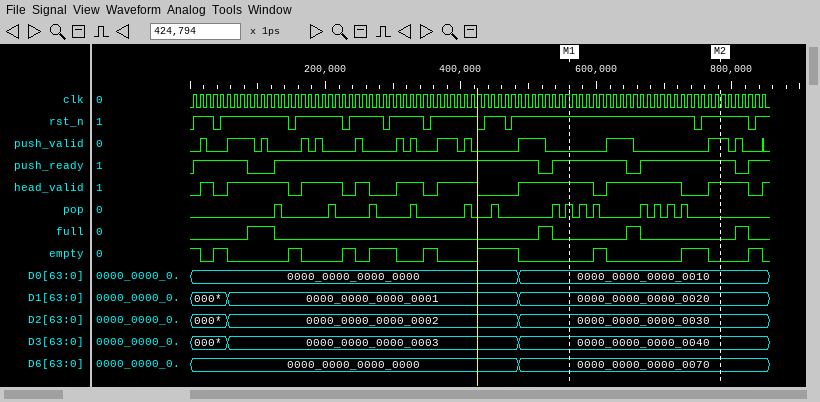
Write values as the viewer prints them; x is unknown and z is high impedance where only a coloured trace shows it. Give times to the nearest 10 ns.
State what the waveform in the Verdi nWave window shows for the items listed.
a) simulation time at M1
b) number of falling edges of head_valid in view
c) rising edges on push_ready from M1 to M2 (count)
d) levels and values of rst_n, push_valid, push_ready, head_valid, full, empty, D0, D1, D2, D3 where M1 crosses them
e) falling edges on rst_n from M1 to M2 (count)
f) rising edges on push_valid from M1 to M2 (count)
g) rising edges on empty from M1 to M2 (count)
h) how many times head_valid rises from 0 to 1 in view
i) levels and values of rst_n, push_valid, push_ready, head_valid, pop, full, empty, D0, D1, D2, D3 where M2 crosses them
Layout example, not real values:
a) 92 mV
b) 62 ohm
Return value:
a) 560 ns
b) 9
c) 1
d) rst_n=1, push_valid=0, push_ready=1, head_valid=1, full=0, empty=0, D0=0000_0000_0000_0010, D1=0000_0000_0000_0020, D2=0000_0000_0000_0030, D3=0000_0000_0000_0040
e) 1
f) 2
g) 2
h) 10
i) rst_n=1, push_valid=1, push_ready=1, head_valid=1, pop=0, full=0, empty=0, D0=0000_0000_0000_0010, D1=0000_0000_0000_0020, D2=0000_0000_0000_0030, D3=0000_0000_0000_0040
